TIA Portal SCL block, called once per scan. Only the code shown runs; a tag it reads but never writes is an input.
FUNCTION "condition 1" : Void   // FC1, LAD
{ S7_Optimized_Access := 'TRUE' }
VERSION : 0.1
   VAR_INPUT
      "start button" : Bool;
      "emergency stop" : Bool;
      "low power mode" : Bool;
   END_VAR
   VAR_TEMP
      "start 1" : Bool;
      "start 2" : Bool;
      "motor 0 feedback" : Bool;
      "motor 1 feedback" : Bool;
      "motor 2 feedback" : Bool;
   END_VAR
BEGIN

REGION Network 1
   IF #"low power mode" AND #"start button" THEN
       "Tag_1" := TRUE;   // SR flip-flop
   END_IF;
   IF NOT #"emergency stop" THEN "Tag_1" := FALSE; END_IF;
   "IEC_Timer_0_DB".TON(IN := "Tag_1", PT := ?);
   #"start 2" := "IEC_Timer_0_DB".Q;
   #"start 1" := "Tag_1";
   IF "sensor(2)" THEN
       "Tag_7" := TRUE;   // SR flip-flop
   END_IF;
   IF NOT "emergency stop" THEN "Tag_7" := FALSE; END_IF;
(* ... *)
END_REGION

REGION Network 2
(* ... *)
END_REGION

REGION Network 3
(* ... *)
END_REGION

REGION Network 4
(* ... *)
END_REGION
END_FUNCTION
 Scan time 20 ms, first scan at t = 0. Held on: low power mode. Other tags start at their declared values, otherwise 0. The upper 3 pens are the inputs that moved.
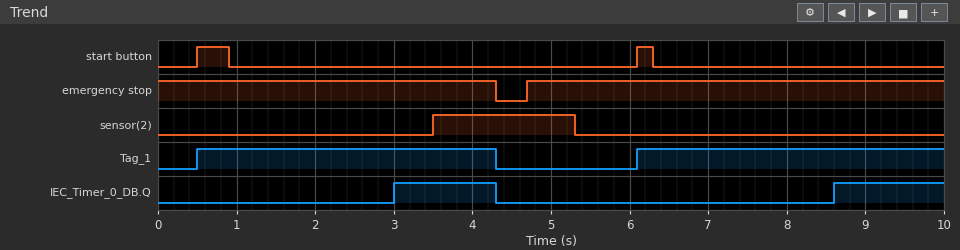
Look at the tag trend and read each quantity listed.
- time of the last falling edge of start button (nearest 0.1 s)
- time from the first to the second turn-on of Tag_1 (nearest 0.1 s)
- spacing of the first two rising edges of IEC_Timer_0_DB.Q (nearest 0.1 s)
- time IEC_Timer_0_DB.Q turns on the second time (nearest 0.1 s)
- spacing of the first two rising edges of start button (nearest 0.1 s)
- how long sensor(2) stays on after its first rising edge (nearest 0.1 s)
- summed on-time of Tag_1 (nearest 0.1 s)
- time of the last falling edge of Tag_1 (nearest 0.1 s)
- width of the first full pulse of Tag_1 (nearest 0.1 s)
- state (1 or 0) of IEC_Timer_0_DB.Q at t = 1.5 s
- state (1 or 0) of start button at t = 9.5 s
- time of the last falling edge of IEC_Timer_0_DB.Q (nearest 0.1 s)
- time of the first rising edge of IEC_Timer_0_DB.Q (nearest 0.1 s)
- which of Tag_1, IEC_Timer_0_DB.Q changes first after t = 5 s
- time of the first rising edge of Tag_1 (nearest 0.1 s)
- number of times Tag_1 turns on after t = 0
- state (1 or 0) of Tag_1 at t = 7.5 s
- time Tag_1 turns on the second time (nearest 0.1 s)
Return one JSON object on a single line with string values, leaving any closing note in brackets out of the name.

{"time of the last falling edge of start button": "6.3 s", "time from the first to the second turn-on of Tag_1": "5.6 s", "spacing of the first two rising edges of IEC_Timer_0_DB.Q": "5.6 s", "time IEC_Timer_0_DB.Q turns on the second time": "8.6 s", "spacing of the first two rising edges of start button": "5.6 s", "how long sensor(2) stays on after its first rising edge": "1.8 s", "summed on-time of Tag_1": "7.7 s", "time of the last falling edge of Tag_1": "4.3 s", "width of the first full pulse of Tag_1": "3.8 s", "state (1 or 0) of IEC_Timer_0_DB.Q at t = 1.5 s": "0", "state (1 or 0) of start button at t = 9.5 s": "0", "time of the last falling edge of IEC_Timer_0_DB.Q": "4.3 s", "time of the first rising edge of IEC_Timer_0_DB.Q": "3.0 s", "which of Tag_1, IEC_Timer_0_DB.Q changes first after t = 5 s": "Tag_1", "time of the first rising edge of Tag_1": "0.5 s", "number of times Tag_1 turns on after t = 0": "2", "state (1 or 0) of Tag_1 at t = 7.5 s": "1", "time Tag_1 turns on the second time": "6.1 s"}
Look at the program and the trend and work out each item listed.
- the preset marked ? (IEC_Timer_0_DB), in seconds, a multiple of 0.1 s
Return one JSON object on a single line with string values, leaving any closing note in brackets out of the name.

{"the preset marked ? (IEC_Timer_0_DB), in seconds, a multiple of 0.1 s": "2.5 s"}
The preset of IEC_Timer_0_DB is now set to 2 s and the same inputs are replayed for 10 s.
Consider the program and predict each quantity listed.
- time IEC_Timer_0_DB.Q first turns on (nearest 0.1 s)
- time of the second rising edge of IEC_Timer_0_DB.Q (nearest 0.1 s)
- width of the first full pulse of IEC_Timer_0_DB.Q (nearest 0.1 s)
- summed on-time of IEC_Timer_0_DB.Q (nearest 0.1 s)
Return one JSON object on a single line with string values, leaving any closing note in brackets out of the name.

{"time IEC_Timer_0_DB.Q first turns on": "2.5 s", "time of the second rising edge of IEC_Timer_0_DB.Q": "8.1 s", "width of the first full pulse of IEC_Timer_0_DB.Q": "1.8 s", "summed on-time of IEC_Timer_0_DB.Q": "3.7 s"}
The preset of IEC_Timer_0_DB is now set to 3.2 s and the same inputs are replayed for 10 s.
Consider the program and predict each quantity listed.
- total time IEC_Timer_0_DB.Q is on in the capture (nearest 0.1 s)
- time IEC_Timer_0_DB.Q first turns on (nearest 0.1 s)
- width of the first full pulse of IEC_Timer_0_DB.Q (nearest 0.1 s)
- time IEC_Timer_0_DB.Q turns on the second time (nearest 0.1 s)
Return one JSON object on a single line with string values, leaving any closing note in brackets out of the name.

{"total time IEC_Timer_0_DB.Q is on in the capture": "1.3 s", "time IEC_Timer_0_DB.Q first turns on": "3.7 s", "width of the first full pulse of IEC_Timer_0_DB.Q": "0.6 s", "time IEC_Timer_0_DB.Q turns on the second time": "9.3 s"}
